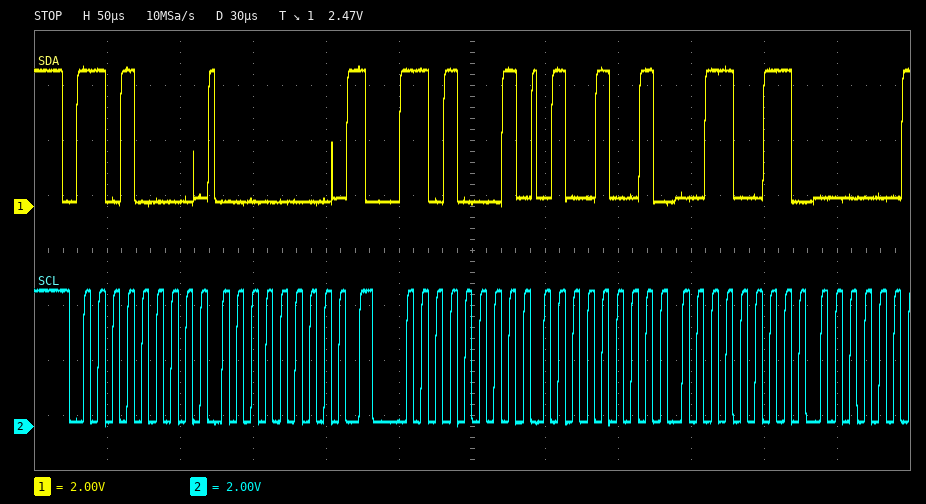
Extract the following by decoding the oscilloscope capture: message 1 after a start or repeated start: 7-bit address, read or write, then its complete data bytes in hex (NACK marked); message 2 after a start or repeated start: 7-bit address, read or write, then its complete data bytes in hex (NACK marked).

0x68 write: 00
0x68 read: 49 33
